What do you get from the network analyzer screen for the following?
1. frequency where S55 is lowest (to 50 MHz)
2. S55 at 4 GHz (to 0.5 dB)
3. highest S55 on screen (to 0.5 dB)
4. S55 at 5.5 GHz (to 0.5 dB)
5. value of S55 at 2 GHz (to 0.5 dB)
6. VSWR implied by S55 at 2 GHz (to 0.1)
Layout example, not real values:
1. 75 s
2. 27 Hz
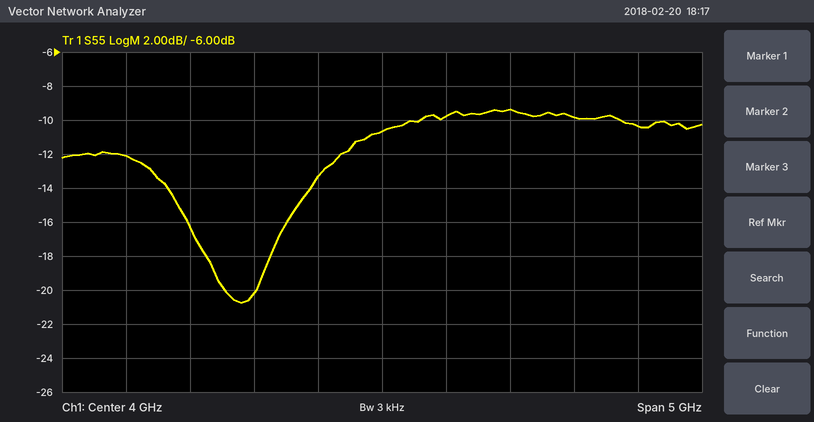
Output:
1. 2.90 GHz
2. -10.5 dB
3. -9.5 dB
4. -10.0 dB
5. -12.0 dB
6. 1.7
